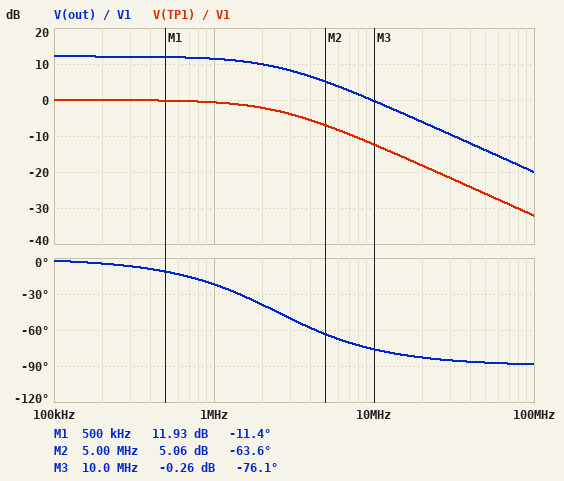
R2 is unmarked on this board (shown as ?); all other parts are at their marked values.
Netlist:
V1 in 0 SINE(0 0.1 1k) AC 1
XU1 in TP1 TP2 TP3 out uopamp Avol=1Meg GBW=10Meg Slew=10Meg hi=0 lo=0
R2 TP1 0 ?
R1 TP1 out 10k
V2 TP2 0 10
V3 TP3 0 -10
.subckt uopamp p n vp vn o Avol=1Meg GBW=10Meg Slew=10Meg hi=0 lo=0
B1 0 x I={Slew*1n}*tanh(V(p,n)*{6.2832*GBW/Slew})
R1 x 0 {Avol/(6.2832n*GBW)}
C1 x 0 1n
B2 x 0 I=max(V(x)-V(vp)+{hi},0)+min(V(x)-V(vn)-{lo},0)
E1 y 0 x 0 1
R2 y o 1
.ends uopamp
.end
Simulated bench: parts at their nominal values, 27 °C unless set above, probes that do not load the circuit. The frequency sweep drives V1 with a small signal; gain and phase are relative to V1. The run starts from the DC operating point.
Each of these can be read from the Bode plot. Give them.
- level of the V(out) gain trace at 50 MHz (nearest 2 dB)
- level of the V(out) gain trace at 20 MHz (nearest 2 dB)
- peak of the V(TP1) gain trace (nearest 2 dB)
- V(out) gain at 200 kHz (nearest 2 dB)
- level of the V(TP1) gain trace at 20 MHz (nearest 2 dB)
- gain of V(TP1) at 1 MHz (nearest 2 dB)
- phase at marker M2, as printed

-14 dB
-6 dB
0 dB
12 dB
-18 dB
0 dB
-63.6 deg
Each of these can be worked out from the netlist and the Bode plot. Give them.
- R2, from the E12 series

3.3 kΩ
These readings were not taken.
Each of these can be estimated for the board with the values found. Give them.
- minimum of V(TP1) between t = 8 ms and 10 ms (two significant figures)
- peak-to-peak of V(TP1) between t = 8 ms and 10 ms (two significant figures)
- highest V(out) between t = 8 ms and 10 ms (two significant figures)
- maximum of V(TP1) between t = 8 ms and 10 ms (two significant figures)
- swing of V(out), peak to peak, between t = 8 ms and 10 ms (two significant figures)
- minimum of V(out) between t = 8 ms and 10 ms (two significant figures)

-100 mV
200 mV
400 mV
100 mV
810 mV
-400 mV
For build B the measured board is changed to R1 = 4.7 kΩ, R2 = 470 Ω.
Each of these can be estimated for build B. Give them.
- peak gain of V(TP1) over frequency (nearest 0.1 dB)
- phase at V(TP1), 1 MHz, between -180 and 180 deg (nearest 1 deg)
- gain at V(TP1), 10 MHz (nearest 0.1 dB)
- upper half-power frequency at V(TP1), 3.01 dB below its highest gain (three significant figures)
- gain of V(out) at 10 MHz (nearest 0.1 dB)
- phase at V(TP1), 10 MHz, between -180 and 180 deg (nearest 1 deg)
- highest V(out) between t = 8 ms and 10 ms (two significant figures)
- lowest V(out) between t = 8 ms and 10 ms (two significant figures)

0 dB
-48 deg
-20.9 dB
909 kHz
0 dB
-85 deg
1.1 V
-1.1 V
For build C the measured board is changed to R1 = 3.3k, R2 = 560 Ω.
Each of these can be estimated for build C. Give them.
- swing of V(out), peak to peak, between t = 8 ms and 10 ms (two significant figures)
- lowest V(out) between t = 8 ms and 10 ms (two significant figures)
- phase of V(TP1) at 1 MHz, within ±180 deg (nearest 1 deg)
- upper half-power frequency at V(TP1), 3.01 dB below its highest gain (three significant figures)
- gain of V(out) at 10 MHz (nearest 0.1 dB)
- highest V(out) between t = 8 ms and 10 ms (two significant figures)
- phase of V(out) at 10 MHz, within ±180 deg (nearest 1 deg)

1.4 V
-690 mV
-35 deg
1.45 MHz
-0.1 dB
690 mV
-82 deg
